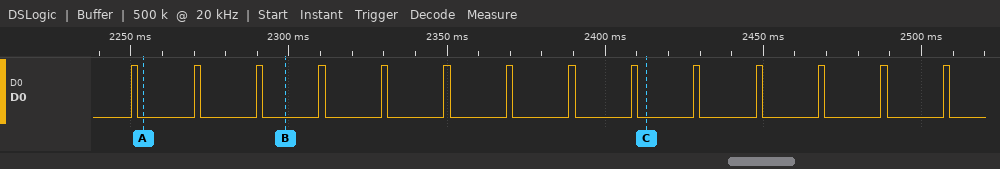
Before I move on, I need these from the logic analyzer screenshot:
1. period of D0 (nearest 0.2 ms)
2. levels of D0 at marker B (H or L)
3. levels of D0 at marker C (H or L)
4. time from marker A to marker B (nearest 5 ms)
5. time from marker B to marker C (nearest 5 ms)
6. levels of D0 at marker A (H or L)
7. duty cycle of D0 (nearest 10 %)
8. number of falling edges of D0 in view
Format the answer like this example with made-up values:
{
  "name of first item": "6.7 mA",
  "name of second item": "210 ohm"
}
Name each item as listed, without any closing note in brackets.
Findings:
{
  "period of D0": "19.8 ms",
  "levels of D0 at marker B": "D0=L",
  "levels of D0 at marker C": "D0=L",
  "time from marker A to marker B": "45 ms",
  "time from marker B to marker C": "115 ms",
  "levels of D0 at marker A": "D0=L",
  "duty cycle of D0": "10 %",
  "number of falling edges of D0 in view": "14"
}
